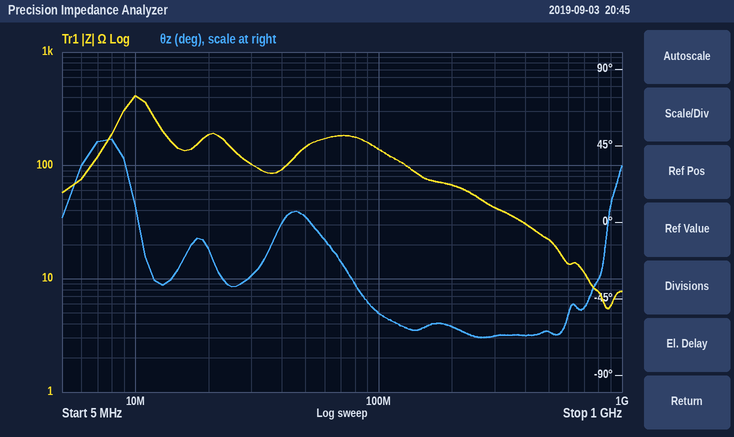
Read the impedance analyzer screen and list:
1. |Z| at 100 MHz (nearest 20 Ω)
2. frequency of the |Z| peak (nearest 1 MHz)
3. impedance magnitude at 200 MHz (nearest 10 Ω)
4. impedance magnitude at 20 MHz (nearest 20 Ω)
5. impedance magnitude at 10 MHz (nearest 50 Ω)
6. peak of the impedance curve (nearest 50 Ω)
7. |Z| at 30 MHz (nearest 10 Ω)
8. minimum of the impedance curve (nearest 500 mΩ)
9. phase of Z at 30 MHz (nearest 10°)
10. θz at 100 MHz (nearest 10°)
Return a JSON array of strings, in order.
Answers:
["140 Ω", "10 MHz", "70 Ω", "180 Ω", "400 Ω", "400 Ω", "100 Ω", "5.5 Ω", "-30°", "-50°"]
